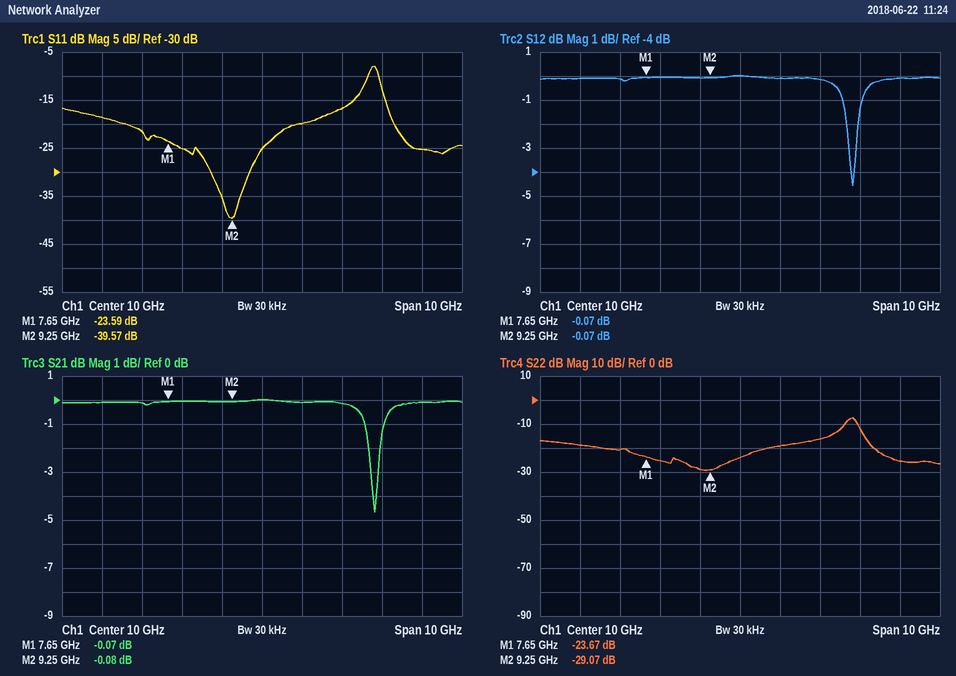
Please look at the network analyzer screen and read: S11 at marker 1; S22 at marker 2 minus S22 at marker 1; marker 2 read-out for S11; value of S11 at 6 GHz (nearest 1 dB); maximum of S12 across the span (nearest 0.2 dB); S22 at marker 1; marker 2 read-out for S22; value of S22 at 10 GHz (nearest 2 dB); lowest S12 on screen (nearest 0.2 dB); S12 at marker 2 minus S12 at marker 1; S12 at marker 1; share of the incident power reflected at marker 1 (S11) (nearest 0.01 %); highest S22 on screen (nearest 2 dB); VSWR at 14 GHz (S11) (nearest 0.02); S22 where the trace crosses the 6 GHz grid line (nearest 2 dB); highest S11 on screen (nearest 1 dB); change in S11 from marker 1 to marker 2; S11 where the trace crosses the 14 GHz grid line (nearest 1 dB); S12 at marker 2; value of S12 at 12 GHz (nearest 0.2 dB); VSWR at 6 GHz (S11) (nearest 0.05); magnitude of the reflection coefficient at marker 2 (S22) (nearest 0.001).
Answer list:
-23.59 dB
-5.40 dB
-39.57 dB
-19 dB
0.0 dB
-23.67 dB
-29.07 dB
-24 dB
-4.6 dB
0.00 dB
-0.07 dB
0.44 %
-8 dB
1.12
-18 dB
-8 dB
-15.98 dB
-25 dB
-0.07 dB
-0.2 dB
1.25
0.035
